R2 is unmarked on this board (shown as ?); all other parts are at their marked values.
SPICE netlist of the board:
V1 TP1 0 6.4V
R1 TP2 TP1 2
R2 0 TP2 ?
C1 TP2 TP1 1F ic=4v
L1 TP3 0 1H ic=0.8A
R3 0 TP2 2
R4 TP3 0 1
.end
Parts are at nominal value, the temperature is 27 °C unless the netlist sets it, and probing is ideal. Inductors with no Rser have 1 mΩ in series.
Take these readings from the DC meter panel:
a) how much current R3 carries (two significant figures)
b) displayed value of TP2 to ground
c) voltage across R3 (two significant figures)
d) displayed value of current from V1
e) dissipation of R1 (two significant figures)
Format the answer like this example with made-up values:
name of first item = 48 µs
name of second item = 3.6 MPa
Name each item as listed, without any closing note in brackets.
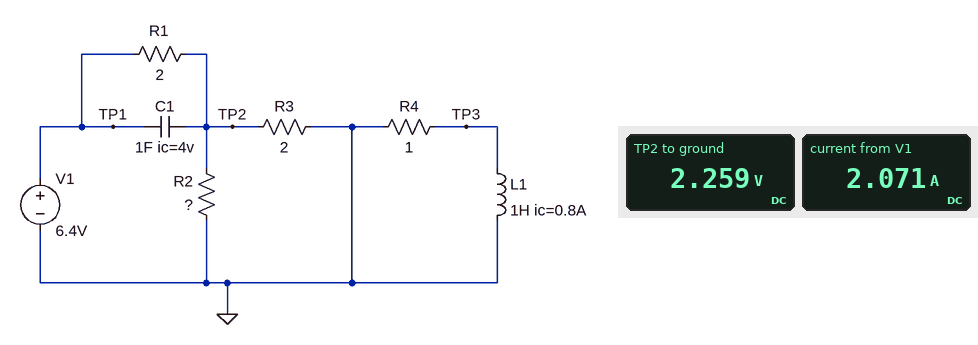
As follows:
how much current R3 carries = 1.1 A
displayed value of TP2 to ground = 2.259 V
voltage across R3 = 2.3 V
displayed value of current from V1 = 2.071 A
dissipation of R1 = 8.6 W
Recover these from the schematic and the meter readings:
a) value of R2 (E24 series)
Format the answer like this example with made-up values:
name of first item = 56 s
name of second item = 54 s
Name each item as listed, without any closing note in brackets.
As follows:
value of R2 = 2.4 Ω
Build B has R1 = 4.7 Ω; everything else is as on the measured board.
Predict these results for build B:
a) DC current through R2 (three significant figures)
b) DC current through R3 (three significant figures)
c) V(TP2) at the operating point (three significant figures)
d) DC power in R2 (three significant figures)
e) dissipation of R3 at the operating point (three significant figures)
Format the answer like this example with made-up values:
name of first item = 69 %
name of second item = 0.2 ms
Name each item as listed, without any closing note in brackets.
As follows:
DC current through R2 = 502 mA
DC current through R3 = 603 mA
V(TP2) at the operating point = 1.21 V
DC power in R2 = 606 mW
dissipation of R3 at the operating point = 727 mW
